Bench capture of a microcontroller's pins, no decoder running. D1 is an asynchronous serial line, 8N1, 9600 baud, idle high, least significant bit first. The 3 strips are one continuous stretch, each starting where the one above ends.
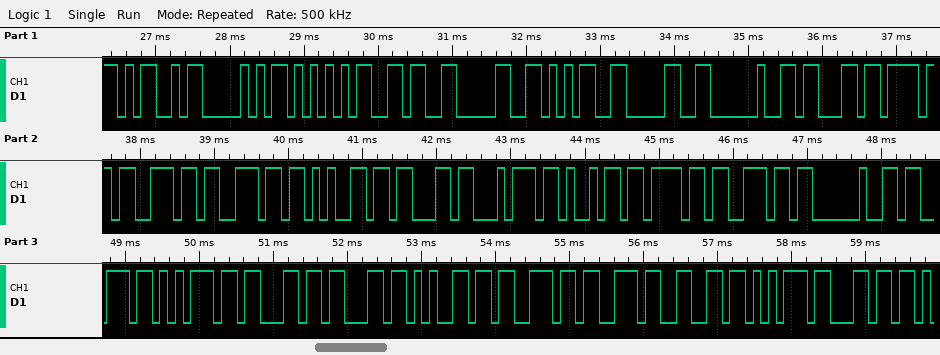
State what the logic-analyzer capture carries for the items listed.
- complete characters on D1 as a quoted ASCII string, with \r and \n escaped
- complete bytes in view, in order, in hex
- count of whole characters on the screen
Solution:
"MPU6050 connection successful"
4D 50 55 36 30 35 30 20 63 6F 6E 6E 65 63 74 69 6F 6E 20 73 75 63 63 65 73 73 66 75 6C
29
